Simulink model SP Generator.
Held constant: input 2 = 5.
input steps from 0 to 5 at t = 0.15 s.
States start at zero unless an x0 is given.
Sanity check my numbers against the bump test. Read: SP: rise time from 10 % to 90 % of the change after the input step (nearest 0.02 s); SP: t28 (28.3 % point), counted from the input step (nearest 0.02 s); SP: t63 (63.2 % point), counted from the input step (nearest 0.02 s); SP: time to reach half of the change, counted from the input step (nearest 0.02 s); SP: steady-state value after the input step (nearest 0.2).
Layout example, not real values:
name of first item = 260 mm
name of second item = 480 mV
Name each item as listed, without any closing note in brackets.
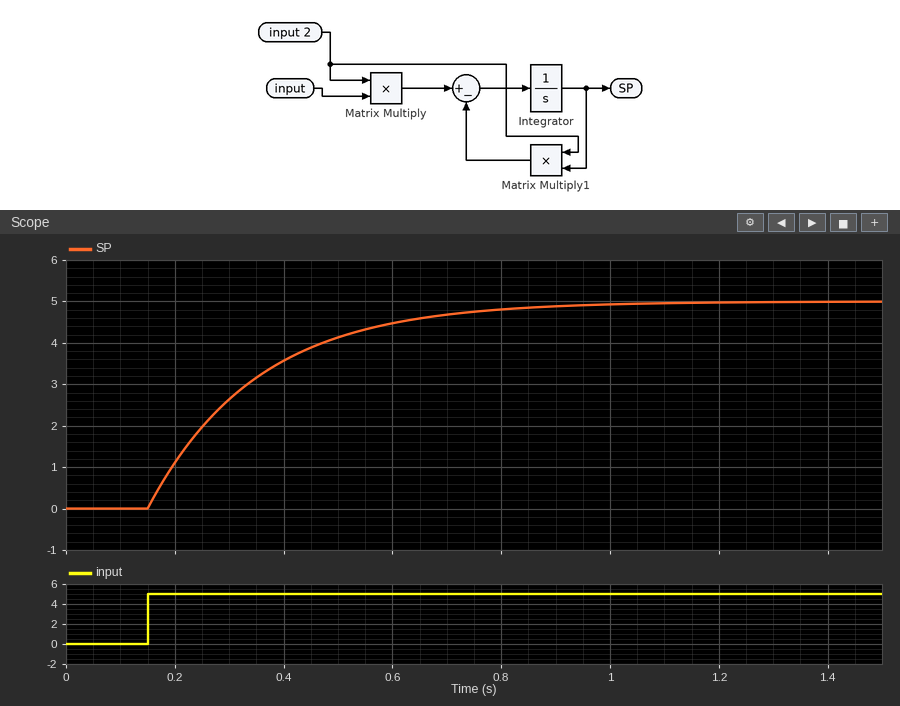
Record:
SP: rise time from 10 % to 90 % of the change after the input step = 0.44 s
SP: t28 (28.3 % point), counted from the input step = 0.06 s
SP: t63 (63.2 % point), counted from the input step = 0.20 s
SP: time to reach half of the change, counted from the input step = 0.14 s
SP: steady-state value after the input step = 5.0
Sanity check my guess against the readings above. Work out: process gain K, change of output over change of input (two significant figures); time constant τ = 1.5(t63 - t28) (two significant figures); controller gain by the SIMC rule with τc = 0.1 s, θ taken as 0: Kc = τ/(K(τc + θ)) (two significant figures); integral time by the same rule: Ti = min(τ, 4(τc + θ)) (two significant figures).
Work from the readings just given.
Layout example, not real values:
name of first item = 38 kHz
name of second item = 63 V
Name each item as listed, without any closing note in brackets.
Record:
process gain K, change of output over change of input = 1.0
time constant τ = 1.5(t63 - t28) = 0.21 s
controller gain by the SIMC rule with τc = 0.1 s, θ taken as 0: Kc = τ/(K(τc + θ)) = 2.1
integral time by the same rule: Ti = min(τ, 4(τc + θ)) = 0.21 s
